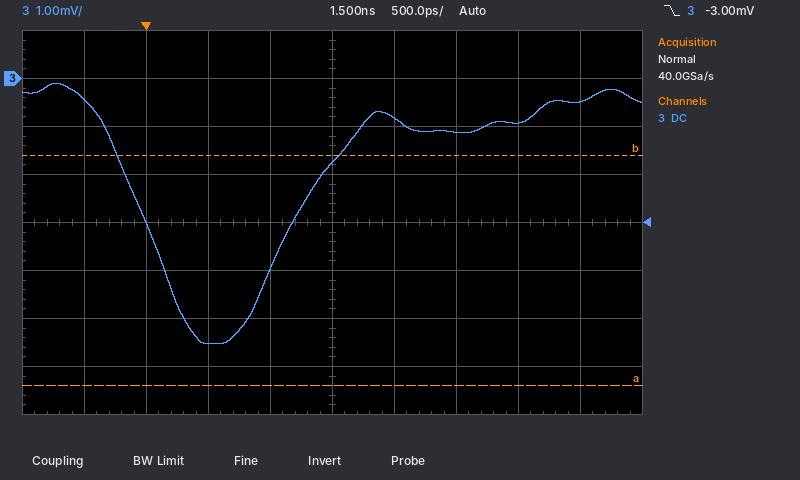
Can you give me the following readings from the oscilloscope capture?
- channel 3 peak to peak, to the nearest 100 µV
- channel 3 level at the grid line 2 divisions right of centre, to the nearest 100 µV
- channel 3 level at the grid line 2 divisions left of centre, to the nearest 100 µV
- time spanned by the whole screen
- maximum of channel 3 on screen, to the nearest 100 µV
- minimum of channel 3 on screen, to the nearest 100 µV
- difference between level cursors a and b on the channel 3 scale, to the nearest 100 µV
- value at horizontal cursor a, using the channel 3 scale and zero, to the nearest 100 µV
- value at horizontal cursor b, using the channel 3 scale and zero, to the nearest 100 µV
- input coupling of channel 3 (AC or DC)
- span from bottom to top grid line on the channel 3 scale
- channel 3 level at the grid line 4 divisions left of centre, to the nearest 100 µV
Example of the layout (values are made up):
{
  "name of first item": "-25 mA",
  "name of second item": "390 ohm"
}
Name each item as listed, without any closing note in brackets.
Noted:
{
  "channel 3 peak to peak, to the nearest 100 µV": "5.4 mV",
  "channel 3 level at the grid line 2 divisions right of centre, to the nearest 100 µV": "-1.1 mV",
  "channel 3 level at the grid line 2 divisions left of centre, to the nearest 100 µV": "-5.5 mV",
  "time spanned by the whole screen": "5 ns",
  "maximum of channel 3 on screen, to the nearest 100 µV": "-100 µV",
  "minimum of channel 3 on screen, to the nearest 100 µV": "-5.5 mV",
  "difference between level cursors a and b on the channel 3 scale, to the nearest 100 µV": "4.8 mV",
  "value at horizontal cursor a, using the channel 3 scale and zero, to the nearest 100 µV": "-6.4 mV",
  "value at horizontal cursor b, using the channel 3 scale and zero, to the nearest 100 µV": "-1.6 mV",
  "input coupling of channel 3": "DC",
  "span from bottom to top grid line on the channel 3 scale": "8 mV",
  "channel 3 level at the grid line 4 divisions left of centre, to the nearest 100 µV": "-400 µV"
}
